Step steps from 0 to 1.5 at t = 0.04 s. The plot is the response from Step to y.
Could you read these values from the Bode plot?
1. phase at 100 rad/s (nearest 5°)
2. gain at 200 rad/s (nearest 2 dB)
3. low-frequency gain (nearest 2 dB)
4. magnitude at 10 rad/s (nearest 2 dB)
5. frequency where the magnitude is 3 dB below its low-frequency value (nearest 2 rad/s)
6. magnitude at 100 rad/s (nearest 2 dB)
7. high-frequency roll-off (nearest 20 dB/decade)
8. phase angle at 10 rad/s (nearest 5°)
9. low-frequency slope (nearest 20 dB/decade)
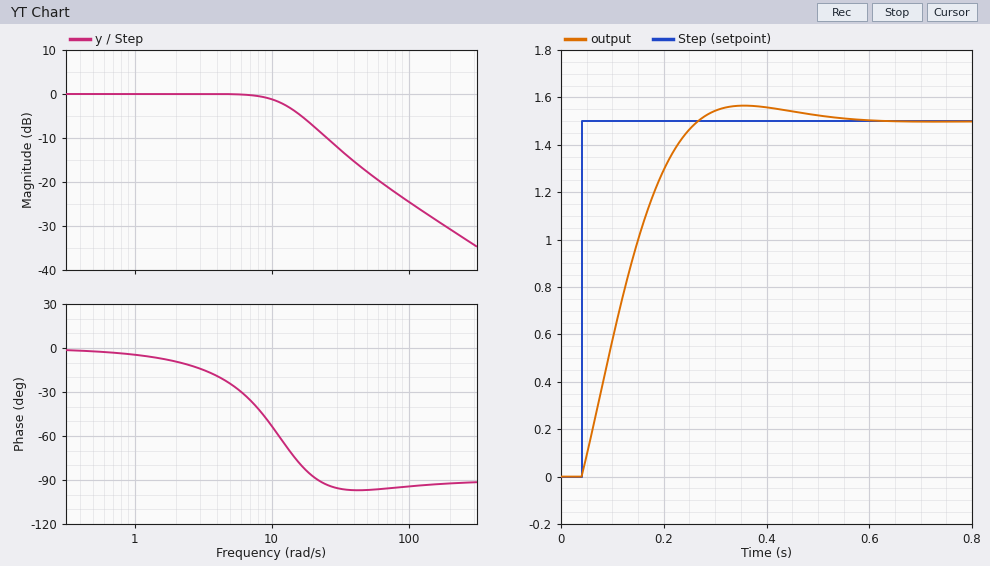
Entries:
-95°
-30 dB
0 dB
-2 dB
14 rad/s
-24 dB
-20 dB/decade
-55°
0 dB/decade
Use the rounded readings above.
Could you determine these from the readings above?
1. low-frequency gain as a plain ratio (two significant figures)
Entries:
1.0
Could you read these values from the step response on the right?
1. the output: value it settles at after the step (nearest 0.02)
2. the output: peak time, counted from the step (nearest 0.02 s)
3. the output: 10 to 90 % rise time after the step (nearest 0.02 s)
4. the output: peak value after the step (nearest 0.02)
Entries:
1.50
0.32 s
0.16 s
1.56
